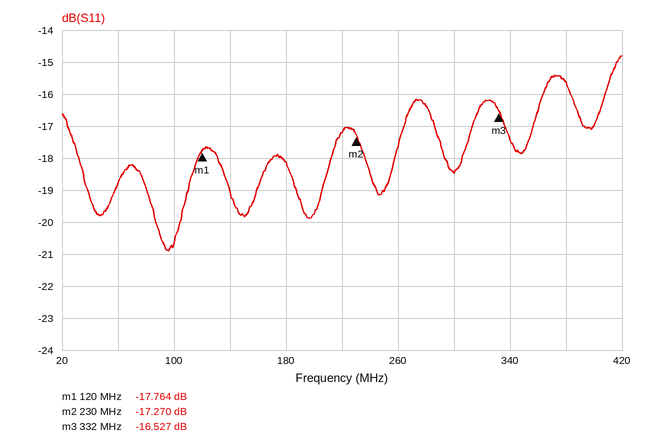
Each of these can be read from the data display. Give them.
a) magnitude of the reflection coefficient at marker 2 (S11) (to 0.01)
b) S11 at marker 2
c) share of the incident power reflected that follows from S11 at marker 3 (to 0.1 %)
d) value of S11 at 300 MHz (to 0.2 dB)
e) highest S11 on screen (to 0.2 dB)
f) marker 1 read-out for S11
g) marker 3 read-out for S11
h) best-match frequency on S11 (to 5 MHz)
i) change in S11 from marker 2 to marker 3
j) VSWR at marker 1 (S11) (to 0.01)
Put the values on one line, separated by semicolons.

0.14; -17.270 dB; 2.2 %; -18.4 dB; -14.8 dB; -17.764 dB; -16.527 dB; 95 MHz; 0.743 dB; 1.30
